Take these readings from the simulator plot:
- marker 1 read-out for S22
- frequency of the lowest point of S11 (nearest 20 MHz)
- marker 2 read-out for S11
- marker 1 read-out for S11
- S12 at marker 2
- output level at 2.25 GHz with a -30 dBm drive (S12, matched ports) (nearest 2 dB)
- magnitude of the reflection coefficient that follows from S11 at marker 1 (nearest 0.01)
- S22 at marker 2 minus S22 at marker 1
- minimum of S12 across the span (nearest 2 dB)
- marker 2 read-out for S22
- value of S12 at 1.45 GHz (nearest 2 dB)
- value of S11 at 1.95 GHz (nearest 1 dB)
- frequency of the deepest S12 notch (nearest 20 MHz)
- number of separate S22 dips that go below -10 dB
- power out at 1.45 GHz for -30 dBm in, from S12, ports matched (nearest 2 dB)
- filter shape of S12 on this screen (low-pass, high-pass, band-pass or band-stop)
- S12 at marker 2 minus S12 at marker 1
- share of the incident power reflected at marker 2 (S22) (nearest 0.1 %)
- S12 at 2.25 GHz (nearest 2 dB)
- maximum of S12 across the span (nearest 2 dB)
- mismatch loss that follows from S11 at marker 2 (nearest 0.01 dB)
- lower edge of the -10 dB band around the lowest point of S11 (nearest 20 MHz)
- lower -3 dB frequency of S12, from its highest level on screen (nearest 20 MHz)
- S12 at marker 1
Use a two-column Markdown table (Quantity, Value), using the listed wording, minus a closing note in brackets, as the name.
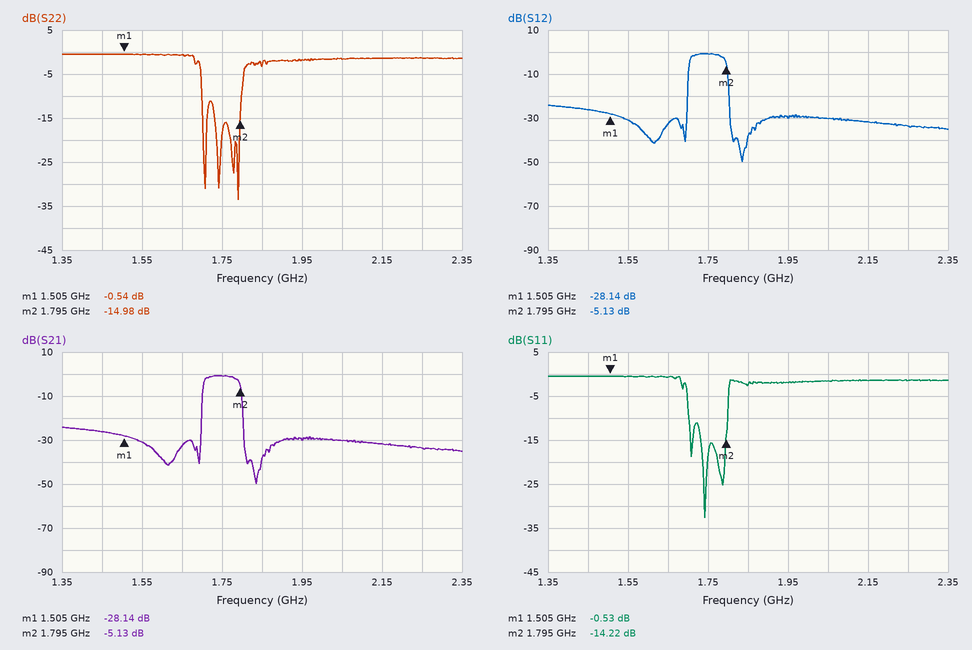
| Quantity | Value |
|---|---|
| marker 1 read-out for S22 | -0.54 dB |
| frequency of the lowest point of S11 | 1.74 GHz |
| marker 2 read-out for S11 | -14.22 dB |
| marker 1 read-out for S11 | -0.53 dB |
| S12 at marker 2 | -5.13 dB |
| output level at 2.25 GHz with a -30 dBm drive (S12, matched ports) | -64 dBm |
| magnitude of the reflection coefficient that follows from S11 at marker 1 | 0.94 |
| S22 at marker 2 minus S22 at marker 1 | -14.44 dB |
| minimum of S12 across the span | -50 dB |
| marker 2 read-out for S22 | -14.98 dB |
| value of S12 at 1.45 GHz | -26 dB |
| value of S11 at 1.95 GHz | -2 dB |
| frequency of the deepest S12 notch | 1.84 GHz |
| number of separate S22 dips that go below -10 dB | 4 |
| power out at 1.45 GHz for -30 dBm in, from S12, ports matched | -56 dBm |
| filter shape of S12 on this screen | band-pass |
| S12 at marker 2 minus S12 at marker 1 | 23.01 dB |
| share of the incident power reflected at marker 2 (S22) | 3.2 % |
| S12 at 2.25 GHz | -34 dB |
| maximum of S12 across the span | 0 dB |
| mismatch loss that follows from S11 at marker 2 | 0.17 dB |
| lower edge of the -10 dB band around the lowest point of S11 | 1.70 GHz |
| lower -3 dB frequency of S12, from its highest level on screen | 1.70 GHz |
| S12 at marker 1 | -28.14 dB |
